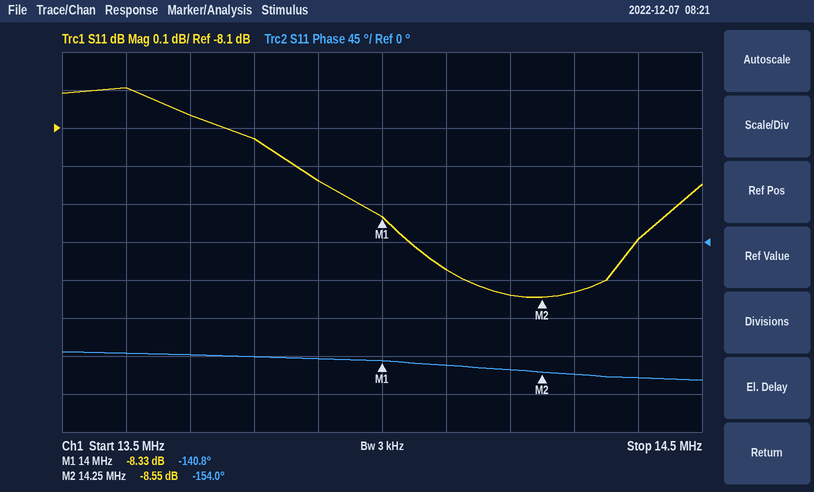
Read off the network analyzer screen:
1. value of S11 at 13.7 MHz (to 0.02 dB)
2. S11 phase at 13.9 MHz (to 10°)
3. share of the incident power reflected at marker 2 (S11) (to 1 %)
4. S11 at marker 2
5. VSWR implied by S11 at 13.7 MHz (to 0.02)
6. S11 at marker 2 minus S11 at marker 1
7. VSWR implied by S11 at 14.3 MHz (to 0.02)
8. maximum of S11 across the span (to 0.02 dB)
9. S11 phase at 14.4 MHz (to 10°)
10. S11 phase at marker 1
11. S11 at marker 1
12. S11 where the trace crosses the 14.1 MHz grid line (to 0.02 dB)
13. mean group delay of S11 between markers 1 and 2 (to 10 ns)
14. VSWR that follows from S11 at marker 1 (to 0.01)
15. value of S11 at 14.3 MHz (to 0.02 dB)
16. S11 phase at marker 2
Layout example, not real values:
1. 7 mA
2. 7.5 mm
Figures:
1. -8.06 dB
2. -140°
3. 14 %
4. -8.55 dB
5. 2.30
6. -0.22 dB
7. 2.20
8. -8.00 dB
9. -160°
10. -140.8°
11. -8.33 dB
12. -8.48 dB
13. 150 ns
14. 2.24
15. -8.54 dB
16. -154.0°
